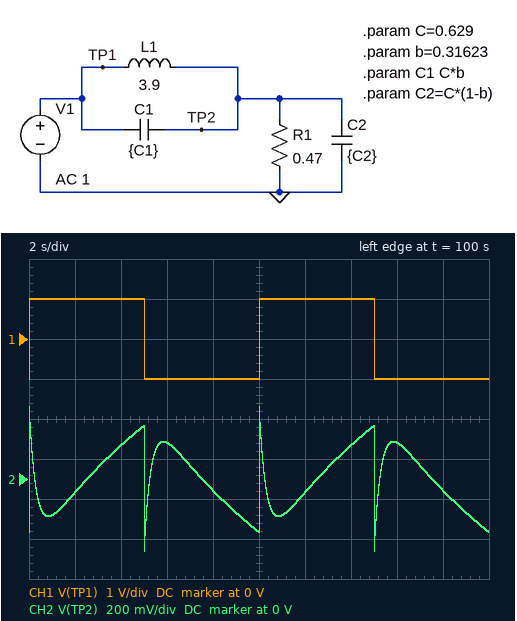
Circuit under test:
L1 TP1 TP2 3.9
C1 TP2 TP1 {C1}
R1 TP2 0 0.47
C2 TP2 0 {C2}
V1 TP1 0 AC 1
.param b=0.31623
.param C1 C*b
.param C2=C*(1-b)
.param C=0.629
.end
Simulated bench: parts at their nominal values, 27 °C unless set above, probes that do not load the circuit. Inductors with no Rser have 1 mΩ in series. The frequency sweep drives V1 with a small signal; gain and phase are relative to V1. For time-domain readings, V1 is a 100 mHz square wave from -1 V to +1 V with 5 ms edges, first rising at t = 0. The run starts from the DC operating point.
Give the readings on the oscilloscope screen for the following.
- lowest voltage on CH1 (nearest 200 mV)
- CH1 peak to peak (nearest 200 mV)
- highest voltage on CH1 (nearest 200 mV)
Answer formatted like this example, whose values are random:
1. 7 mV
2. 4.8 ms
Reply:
1. -1.0 V
2. 2.0 V
3. 1.0 V
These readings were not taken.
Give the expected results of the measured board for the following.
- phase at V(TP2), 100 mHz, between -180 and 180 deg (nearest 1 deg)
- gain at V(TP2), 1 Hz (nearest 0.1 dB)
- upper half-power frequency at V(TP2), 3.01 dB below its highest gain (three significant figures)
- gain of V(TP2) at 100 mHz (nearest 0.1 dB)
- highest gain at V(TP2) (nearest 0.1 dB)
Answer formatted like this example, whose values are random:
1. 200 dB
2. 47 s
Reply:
1. -90 deg
2. -11.3 dB
3. 19.5 mHz
4. -17.5 dB
5. 0 dB
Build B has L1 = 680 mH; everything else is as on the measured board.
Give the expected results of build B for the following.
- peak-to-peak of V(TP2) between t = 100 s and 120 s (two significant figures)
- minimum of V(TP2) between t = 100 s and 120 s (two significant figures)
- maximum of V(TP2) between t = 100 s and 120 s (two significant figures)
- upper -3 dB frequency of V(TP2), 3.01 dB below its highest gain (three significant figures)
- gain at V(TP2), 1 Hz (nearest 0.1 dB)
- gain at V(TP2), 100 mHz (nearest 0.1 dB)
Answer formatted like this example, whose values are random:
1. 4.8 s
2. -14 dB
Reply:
1. 1.9 V
2. -970 mV
3. 970 mV
4. 117 mHz
5. -12.5 dB
6. -2.3 dB
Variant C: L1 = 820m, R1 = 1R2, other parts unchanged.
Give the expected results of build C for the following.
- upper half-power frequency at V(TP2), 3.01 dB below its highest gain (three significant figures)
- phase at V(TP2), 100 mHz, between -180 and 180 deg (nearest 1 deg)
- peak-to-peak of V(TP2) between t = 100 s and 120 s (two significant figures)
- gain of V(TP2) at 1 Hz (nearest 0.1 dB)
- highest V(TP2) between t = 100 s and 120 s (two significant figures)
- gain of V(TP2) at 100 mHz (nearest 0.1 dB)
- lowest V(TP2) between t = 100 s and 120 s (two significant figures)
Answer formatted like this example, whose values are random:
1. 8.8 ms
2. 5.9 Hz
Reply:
1. 219 mHz
2. -28 deg
3. 2.5 V
4. -11.2 dB
5. 1.3 V
6. 0.3 dB
7. -1.3 V
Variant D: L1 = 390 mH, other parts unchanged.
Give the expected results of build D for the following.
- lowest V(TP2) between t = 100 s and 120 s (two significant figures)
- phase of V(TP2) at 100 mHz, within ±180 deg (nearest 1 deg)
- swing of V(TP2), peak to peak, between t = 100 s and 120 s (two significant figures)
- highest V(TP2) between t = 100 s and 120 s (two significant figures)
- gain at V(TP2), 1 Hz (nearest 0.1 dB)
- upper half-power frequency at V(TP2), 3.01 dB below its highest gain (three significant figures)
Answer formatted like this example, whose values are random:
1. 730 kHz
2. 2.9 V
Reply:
1. -1.0 V
2. -30 deg
3. 2.0 V
4. 1.0 V
5. -13.8 dB
6. 207 mHz
